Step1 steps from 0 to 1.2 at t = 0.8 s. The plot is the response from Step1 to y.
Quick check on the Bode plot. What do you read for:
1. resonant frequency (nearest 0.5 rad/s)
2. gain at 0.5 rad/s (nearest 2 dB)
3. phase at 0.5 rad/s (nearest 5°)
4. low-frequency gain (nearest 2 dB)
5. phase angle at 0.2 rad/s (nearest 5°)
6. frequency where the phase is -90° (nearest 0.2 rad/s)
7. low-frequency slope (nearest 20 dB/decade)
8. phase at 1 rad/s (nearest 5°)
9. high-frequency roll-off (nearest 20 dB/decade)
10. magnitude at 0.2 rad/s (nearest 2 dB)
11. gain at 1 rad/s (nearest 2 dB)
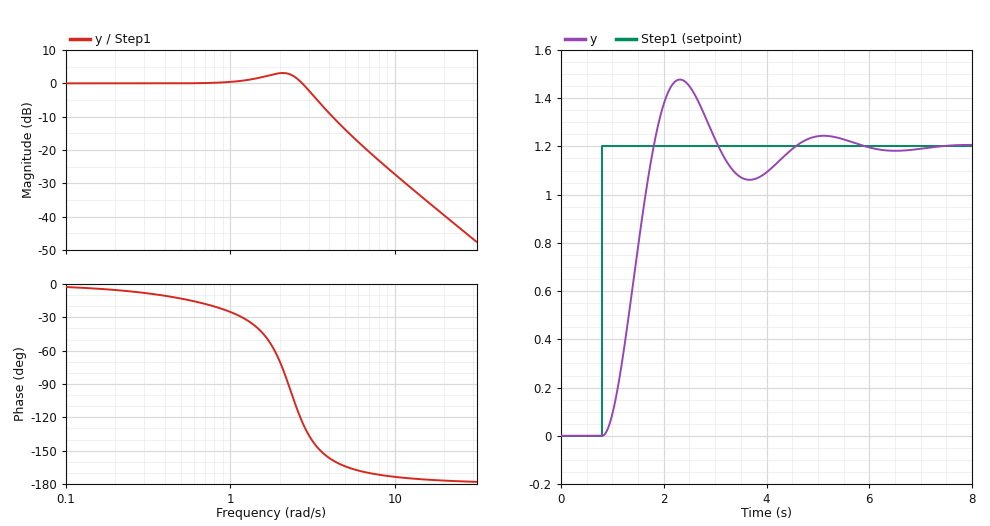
2.0 rad/s
0 dB
-15°
0 dB
-5°
2.2 rad/s
0 dB/decade
-25°
-40 dB/decade
0 dB
0 dB
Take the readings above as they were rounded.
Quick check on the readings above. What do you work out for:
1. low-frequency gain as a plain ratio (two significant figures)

1.0
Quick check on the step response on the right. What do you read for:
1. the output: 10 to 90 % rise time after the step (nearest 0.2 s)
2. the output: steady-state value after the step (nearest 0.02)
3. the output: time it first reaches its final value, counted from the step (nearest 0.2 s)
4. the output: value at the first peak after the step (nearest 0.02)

0.6 s
1.20
1.0 s
1.48
